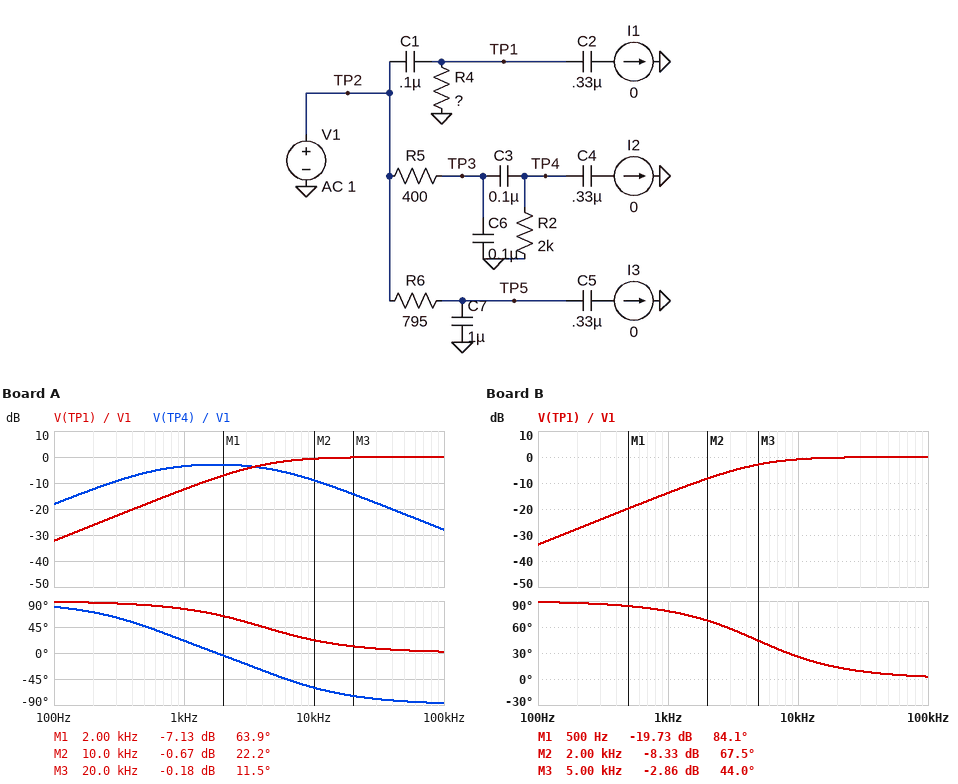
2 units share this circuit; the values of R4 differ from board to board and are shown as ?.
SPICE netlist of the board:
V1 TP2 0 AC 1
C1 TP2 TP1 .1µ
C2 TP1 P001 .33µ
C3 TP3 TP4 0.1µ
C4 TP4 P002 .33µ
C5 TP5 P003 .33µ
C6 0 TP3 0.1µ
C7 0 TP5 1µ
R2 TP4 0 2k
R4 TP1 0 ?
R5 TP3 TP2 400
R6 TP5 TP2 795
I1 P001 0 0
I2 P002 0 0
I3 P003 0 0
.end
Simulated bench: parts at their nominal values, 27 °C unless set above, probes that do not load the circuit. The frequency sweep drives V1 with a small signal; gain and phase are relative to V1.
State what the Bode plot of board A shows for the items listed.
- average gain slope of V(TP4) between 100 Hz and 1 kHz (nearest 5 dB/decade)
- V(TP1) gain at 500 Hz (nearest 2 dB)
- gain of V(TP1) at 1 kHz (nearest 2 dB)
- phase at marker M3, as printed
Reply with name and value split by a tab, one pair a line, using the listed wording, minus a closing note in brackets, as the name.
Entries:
average gain slope of V(TP4) between 100 Hz and 1 kHz	15 dB/decade
V(TP1) gain at 500 Hz	-18 dB
gain of V(TP1) at 1 kHz	-12 dB
phase at marker M3, as printed	11.5 deg
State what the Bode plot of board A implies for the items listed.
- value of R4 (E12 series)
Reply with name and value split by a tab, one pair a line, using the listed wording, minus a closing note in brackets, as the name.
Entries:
value of R4	390 Ω
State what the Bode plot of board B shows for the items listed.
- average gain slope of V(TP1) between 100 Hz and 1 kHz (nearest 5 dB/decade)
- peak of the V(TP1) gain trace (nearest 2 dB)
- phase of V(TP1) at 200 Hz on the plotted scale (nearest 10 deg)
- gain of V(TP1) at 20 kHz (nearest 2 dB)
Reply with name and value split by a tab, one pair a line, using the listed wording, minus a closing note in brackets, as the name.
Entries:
average gain slope of V(TP1) between 100 Hz and 1 kHz	20 dB/decade
peak of the V(TP1) gain trace	0 dB
phase of V(TP1) at 200 Hz on the plotted scale	90 deg
gain of V(TP1) at 20 kHz	0 dB
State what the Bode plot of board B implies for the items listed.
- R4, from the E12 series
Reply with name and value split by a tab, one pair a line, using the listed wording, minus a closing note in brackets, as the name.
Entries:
R4, from the E12 series	330 Ω
